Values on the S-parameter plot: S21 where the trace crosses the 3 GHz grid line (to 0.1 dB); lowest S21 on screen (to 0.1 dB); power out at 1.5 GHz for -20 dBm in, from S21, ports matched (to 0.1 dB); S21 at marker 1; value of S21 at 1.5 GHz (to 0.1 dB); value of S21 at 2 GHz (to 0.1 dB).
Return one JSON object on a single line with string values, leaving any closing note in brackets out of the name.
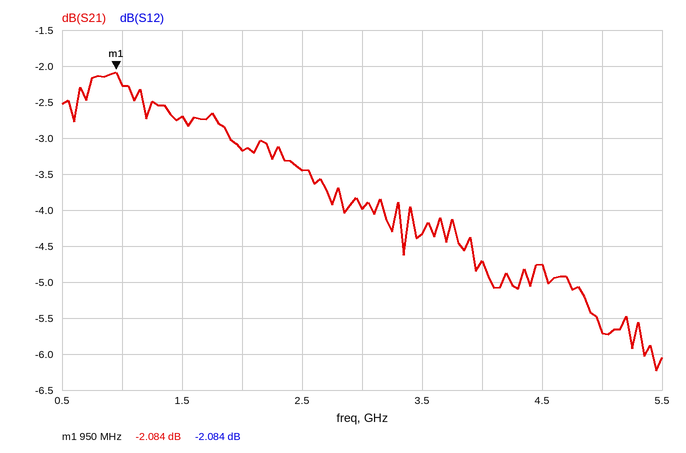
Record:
{"S21 where the trace crosses the 3 GHz grid line": "-4.0 dB", "lowest S21 on screen": "-6.2 dB", "power out at 1.5 GHz for -20 dBm in, from S21, ports matched": "-22.7 dBm", "S21 at marker 1": "-2.084 dB", "value of S21 at 1.5 GHz": "-2.7 dB", "value of S21 at 2 GHz": "-3.2 dB"}
